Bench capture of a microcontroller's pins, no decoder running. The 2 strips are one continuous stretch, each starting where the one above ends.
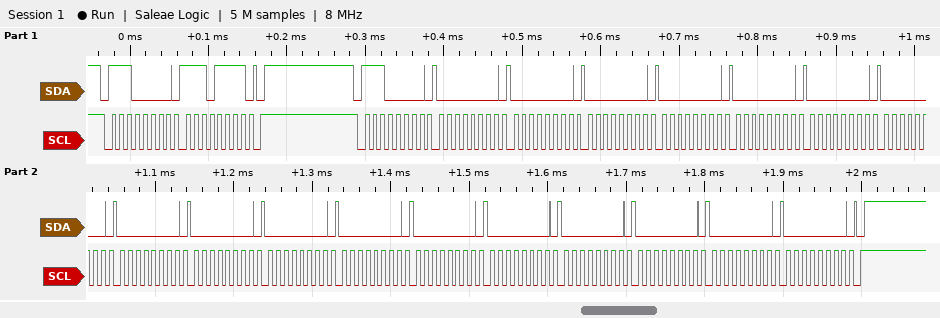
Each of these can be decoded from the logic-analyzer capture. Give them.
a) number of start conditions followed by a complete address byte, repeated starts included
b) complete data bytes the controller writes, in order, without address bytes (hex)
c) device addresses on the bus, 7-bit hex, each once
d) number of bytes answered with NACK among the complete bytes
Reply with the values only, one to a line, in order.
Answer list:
2
EF 00 00 00 00 00 00 00 00 00 00 00 00 00 00 00 00 00
0x70
0
